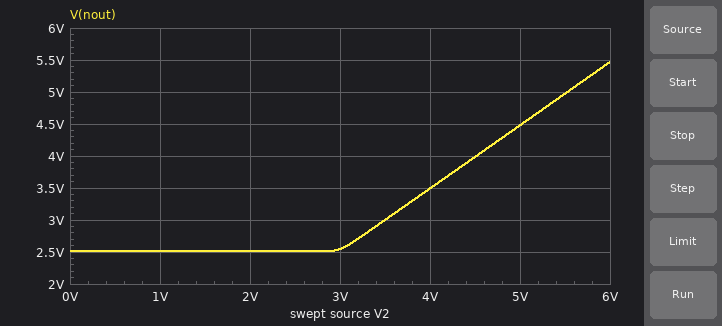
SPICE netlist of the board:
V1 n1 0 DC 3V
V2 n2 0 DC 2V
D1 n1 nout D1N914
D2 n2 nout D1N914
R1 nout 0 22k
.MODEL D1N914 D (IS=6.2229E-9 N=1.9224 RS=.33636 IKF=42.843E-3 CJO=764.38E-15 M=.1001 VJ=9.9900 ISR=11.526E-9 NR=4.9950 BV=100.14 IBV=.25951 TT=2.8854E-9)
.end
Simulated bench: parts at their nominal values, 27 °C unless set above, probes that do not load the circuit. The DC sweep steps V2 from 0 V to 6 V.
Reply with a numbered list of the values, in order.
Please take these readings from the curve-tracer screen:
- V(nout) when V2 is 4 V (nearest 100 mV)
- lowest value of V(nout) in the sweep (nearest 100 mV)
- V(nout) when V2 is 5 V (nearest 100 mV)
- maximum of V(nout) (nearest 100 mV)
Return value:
1. 3.5 V
2. 2.5 V
3. 4.5 V
4. 5.5 V
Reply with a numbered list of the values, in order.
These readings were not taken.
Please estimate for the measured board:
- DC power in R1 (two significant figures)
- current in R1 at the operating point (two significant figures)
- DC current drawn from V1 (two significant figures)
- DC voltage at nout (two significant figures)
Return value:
1. 290 µW
2. 110 µA
3. 110 µA
4. 2.5 V
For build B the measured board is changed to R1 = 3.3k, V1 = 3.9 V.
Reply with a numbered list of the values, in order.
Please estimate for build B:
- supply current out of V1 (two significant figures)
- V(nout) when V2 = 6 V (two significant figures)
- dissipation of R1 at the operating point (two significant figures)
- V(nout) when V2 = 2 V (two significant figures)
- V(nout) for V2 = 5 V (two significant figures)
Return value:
1. 1.0 mA
2. 5.4 V
3. 3.3 mW
4. 3.3 V
5. 4.4 V
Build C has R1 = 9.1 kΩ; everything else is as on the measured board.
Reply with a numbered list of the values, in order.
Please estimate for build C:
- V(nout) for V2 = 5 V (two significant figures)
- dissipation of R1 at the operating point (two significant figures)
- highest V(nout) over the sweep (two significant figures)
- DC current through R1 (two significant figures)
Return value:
1. 4.4 V
2. 670 µW
3. 5.4 V
4. 270 µA
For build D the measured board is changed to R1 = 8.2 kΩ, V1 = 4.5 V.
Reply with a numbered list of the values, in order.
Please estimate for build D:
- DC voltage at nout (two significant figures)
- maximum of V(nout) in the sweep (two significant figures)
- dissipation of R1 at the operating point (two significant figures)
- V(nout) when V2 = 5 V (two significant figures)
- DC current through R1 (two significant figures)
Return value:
1. 3.9 V
2. 5.4 V
3. 1.9 mW
4. 4.4 V
5. 480 µA
